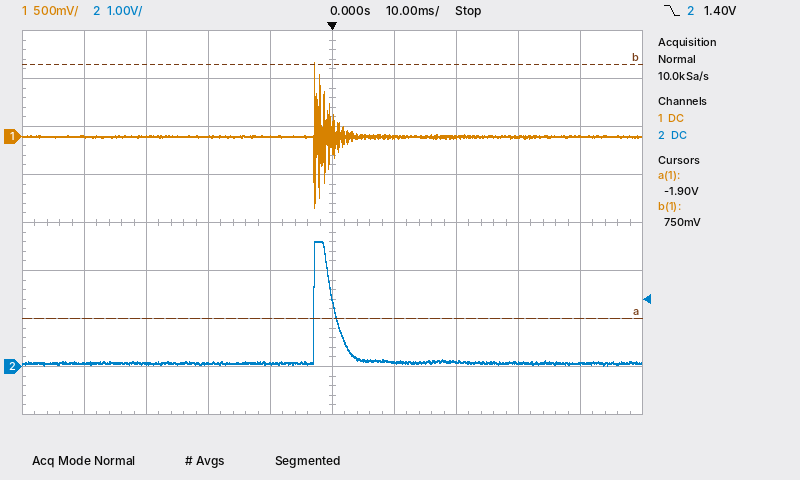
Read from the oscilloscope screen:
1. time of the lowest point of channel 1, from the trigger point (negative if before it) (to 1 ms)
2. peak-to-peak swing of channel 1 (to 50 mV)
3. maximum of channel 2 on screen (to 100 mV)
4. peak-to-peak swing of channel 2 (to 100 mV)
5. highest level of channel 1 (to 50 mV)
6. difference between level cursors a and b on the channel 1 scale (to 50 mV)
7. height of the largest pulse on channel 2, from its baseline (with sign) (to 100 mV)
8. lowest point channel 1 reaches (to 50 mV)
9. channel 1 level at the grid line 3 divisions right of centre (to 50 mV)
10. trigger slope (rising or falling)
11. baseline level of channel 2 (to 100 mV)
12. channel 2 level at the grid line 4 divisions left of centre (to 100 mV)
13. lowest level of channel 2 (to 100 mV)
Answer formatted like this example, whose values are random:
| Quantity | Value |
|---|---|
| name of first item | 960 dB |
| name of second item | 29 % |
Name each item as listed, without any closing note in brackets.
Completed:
| Quantity | Value |
|---|---|
| time of the lowest point of channel 1, from the trigger point (negative if before it) | -3 ms |
| peak-to-peak swing of channel 1 | 1.50 V |
| maximum of channel 2 on screen | 2.6 V |
| peak-to-peak swing of channel 2 | 2.6 V |
| highest level of channel 1 | 750 mV |
| difference between level cursors a and b on the channel 1 scale | 2.65 V |
| height of the largest pulse on channel 2, from its baseline (with sign) | +2.5 V |
| lowest point channel 1 reaches | -750 mV |
| channel 1 level at the grid line 3 divisions right of centre | 0 mV |
| trigger slope | falling |
| baseline level of channel 2 | 100 mV |
| channel 2 level at the grid line 4 divisions left of centre | 100 mV |
| lowest level of channel 2 | 0.0 V |
